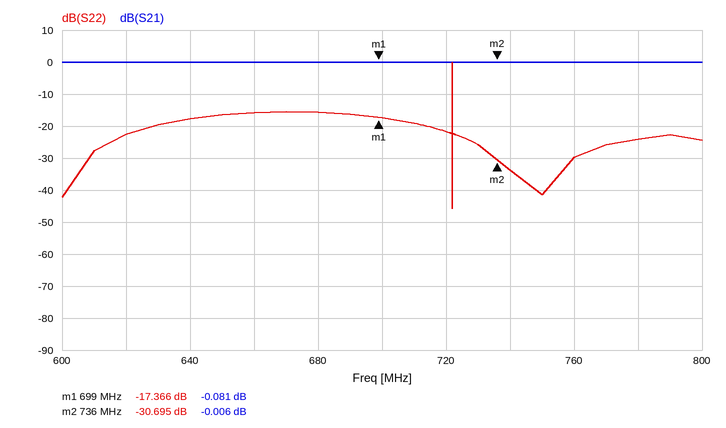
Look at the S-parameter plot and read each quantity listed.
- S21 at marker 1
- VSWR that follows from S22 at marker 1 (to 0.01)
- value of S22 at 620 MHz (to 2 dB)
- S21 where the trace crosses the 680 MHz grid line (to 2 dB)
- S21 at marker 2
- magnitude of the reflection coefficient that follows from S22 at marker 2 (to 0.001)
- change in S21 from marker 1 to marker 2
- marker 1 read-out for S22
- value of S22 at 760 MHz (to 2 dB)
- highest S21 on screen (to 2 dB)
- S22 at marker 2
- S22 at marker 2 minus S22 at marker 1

-0.081 dB
1.31
-22 dB
0 dB
-0.006 dB
0.029
0.075 dB
-17.366 dB
-30 dB
0 dB
-30.695 dB
-13.329 dB
